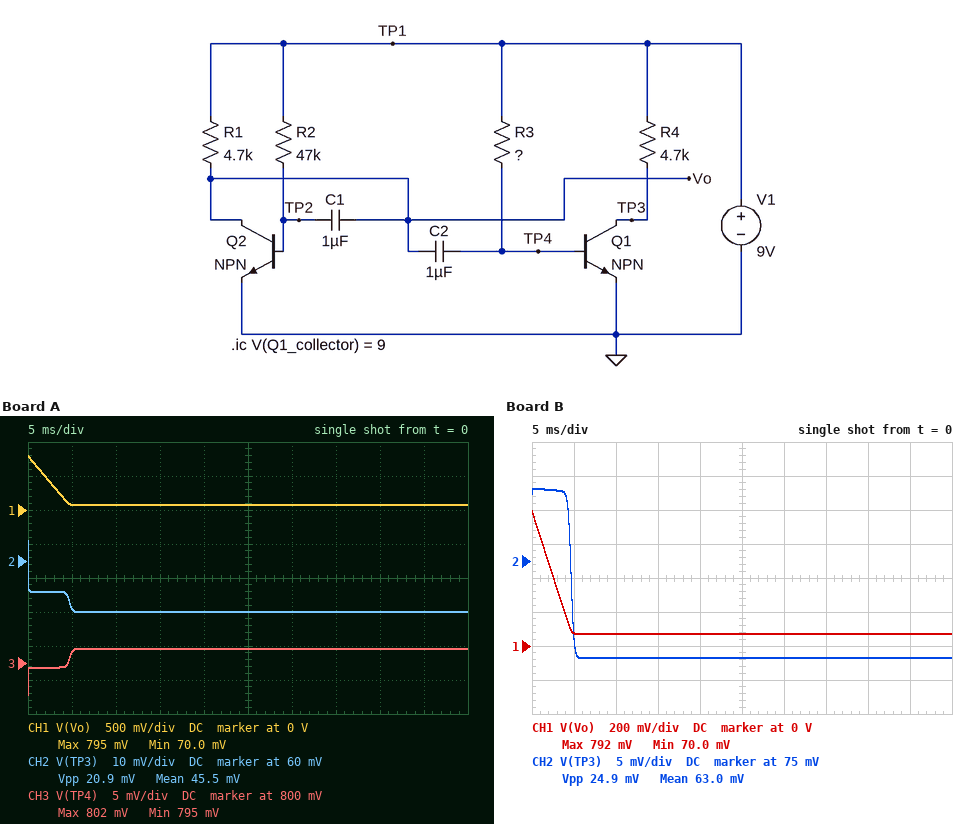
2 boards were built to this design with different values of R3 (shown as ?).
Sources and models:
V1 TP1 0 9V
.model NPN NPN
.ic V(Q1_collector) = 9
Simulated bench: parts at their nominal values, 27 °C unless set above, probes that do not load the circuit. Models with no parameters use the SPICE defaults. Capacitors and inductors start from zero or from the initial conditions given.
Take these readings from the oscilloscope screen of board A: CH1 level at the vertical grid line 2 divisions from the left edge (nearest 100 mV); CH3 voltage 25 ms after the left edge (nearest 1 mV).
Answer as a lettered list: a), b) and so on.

a) 100 mV
b) 802 mV
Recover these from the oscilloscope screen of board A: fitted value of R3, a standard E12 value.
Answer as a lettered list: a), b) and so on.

a) 15 kΩ
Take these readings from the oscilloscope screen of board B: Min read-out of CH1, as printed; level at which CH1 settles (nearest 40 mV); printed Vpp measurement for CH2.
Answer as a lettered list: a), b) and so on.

a) 70.0 mV
b) 80 mV
c) 24.9 mV
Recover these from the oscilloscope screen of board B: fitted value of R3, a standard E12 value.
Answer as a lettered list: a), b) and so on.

a) 33 kΩ
